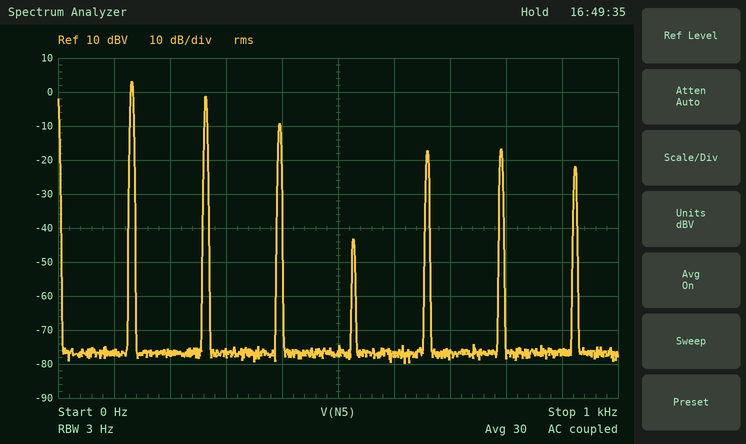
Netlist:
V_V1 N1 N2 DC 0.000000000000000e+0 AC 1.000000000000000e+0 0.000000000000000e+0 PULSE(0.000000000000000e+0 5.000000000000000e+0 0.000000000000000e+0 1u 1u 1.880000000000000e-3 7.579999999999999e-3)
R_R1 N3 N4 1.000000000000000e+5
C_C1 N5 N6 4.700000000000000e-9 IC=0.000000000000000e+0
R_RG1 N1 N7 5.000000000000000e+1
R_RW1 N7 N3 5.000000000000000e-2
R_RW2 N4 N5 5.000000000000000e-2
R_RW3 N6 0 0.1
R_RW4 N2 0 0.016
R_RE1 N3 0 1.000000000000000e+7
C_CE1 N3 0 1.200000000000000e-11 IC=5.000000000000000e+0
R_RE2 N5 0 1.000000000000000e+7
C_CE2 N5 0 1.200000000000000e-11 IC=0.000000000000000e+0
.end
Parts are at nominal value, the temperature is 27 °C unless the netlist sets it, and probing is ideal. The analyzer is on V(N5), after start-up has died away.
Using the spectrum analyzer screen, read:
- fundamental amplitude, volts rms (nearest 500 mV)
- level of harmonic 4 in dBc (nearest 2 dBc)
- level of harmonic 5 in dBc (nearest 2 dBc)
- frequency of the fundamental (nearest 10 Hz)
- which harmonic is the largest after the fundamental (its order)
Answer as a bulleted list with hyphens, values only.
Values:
- 1.5 V
- -46 dBc
- -20 dBc
- 130 Hz
- 2
